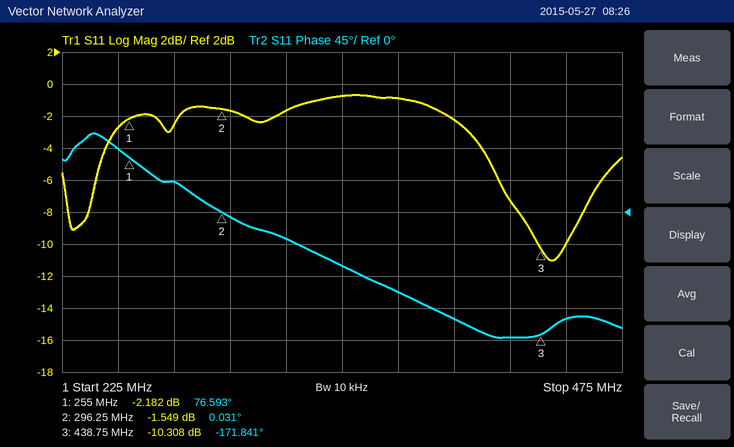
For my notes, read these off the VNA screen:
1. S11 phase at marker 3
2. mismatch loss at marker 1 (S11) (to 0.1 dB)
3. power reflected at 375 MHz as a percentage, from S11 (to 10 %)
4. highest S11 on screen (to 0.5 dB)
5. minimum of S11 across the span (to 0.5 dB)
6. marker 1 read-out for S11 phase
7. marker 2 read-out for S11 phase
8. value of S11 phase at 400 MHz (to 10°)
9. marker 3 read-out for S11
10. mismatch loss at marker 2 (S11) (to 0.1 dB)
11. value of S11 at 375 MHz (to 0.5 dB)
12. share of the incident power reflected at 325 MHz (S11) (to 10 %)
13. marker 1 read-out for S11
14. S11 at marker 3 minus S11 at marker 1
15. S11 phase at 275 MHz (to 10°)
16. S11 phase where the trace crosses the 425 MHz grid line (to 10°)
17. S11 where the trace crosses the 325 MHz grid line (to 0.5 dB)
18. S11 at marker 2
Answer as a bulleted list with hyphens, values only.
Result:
- -171.841°
- 4.0 dB
- 80 %
- -0.5 dB
- -11.0 dB
- 76.593°
- 0.031°
- -150°
- -10.308 dB
- 5.2 dB
- -1.0 dB
- 70 %
- -2.182 dB
- -8.126 dB
- 40°
- -180°
- -1.5 dB
- -1.549 dB
